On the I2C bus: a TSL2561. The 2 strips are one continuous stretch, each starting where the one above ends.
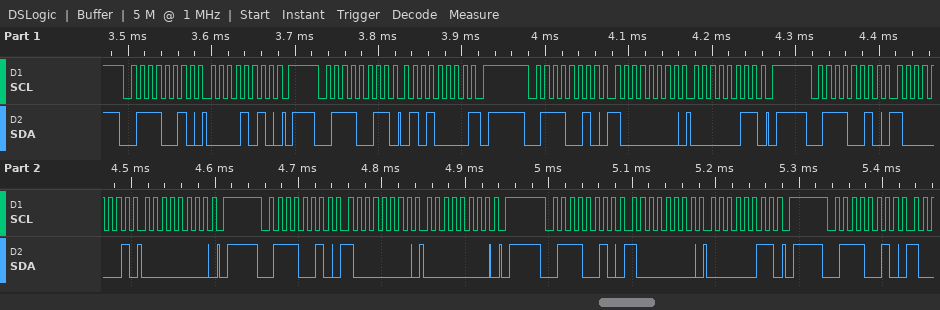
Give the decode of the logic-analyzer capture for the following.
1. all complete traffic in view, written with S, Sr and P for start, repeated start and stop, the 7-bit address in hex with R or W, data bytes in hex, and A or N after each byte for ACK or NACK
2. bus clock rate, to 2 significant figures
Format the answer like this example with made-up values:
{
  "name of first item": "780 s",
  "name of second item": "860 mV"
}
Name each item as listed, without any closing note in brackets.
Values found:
{
  "all complete traffic in view, written with S, Sr and P for start, repeated start and stop, the 7-bit address in hex with R or W, data bytes in hex, and A or N after each byte for ACK or NACK": "S 39W A 0A A P S 39R A 50 N P S 39W A 80 A 03 A P S 39W A 81 A 00 A P S 39W A 80 A 00 A P S 39W A 80 A 03 A P S 39W A",
  "bus clock rate, to 2 significant figures": "100 kHz"
}
